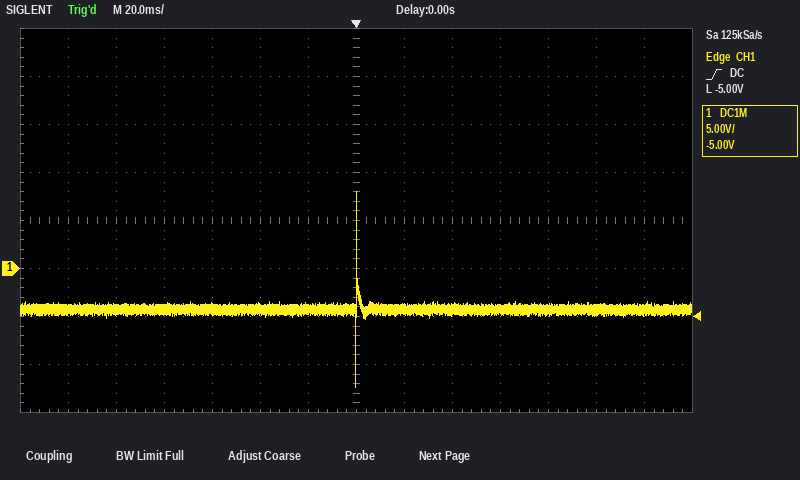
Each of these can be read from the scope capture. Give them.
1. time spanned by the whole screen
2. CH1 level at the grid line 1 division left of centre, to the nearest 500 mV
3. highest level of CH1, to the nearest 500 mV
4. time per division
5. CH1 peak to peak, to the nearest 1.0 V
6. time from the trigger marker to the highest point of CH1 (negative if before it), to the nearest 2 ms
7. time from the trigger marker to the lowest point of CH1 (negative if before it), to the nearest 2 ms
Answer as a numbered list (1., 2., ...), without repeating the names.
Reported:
1. 280 ms
2. -4.0 V
3. 8.0 V
4. 20 ms
5. 20.0 V
6. 0 ms
7. 0 ms
